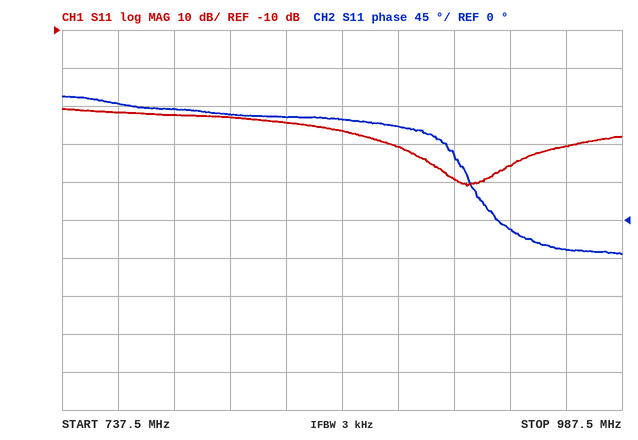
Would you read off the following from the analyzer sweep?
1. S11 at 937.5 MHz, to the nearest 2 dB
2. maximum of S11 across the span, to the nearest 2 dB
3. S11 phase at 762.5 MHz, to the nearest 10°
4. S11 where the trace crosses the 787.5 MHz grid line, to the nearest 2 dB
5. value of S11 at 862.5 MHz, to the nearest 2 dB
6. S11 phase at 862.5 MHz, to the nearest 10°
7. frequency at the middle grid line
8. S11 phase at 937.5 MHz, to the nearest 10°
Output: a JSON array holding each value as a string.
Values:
["-46 dB", "-30 dB", "140°", "-32 dB", "-36 dB", "120°", "862.5 MHz", "-10°"]
